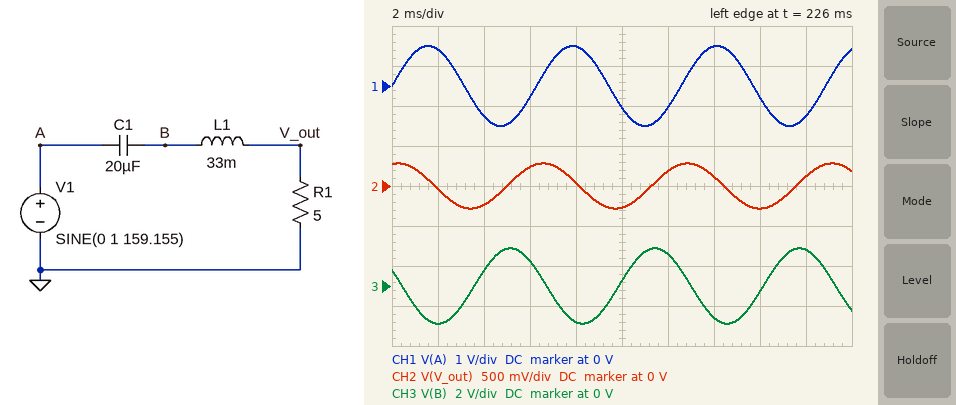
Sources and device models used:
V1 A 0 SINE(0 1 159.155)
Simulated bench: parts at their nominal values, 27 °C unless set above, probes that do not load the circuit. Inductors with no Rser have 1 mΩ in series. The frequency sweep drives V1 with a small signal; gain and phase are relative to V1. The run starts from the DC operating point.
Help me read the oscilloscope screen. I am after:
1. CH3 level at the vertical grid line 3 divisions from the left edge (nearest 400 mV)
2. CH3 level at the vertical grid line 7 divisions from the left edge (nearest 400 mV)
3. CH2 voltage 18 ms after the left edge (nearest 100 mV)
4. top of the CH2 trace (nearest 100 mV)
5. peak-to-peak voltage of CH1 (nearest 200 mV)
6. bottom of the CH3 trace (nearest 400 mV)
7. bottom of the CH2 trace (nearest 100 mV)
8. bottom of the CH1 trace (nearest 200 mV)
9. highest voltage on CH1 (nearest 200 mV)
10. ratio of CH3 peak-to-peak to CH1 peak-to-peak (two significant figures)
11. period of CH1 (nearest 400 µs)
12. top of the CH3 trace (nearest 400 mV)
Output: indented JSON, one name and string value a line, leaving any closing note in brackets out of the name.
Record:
{
  "CH3 level at the vertical grid line 3 divisions from the left edge": "1.2 V",
  "CH3 level at the vertical grid line 7 divisions from the left edge": "-1.6 V",
  "CH2 voltage 18 ms after the left edge": "100 mV",
  "top of the CH2 trace": "300 mV",
  "peak-to-peak voltage of CH1": "2.0 V",
  "bottom of the CH3 trace": "-2.0 V",
  "bottom of the CH2 trace": "-300 mV",
  "bottom of the CH1 trace": "-1.0 V",
  "highest voltage on CH1": "1.0 V",
  "ratio of CH3 peak-to-peak to CH1 peak-to-peak": "1.9",
  "period of CH1": "6.4 ms",
  "top of the CH3 trace": "2.0 V"
}
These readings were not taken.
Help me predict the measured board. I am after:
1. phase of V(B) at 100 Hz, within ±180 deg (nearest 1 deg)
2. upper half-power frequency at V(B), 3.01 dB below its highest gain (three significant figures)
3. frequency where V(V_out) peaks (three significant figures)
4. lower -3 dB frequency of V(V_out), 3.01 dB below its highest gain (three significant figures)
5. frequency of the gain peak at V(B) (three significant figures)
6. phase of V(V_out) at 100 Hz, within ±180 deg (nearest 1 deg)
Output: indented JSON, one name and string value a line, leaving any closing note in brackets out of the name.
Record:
{
  "phase of V(B) at 100 Hz, within ±180 deg": "162 deg",
  "upper half-power frequency at V(B), 3.01 dB below its highest gain": "210 Hz",
  "frequency where V(V_out) peaks": "196 Hz",
  "lower -3 dB frequency of V(V_out), 3.01 dB below its highest gain": "184 Hz",
  "frequency of the gain peak at V(B)": "197 Hz",
  "phase of V(V_out) at 100 Hz, within ±180 deg": "85 deg"
}
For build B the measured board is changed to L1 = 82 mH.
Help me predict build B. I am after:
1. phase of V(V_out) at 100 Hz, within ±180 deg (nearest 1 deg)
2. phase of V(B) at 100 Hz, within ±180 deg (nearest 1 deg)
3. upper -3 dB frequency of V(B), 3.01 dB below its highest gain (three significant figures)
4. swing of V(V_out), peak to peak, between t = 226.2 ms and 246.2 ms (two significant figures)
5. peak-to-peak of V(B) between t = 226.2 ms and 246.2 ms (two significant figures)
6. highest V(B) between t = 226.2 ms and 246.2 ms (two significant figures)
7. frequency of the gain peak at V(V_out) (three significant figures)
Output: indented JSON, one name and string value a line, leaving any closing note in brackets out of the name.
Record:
{
  "phase of V(V_out) at 100 Hz, within ±180 deg": "80 deg",
  "phase of V(B) at 100 Hz, within ±180 deg": "164 deg",
  "upper -3 dB frequency of V(B), 3.01 dB below its highest gain": "130 Hz",
  "swing of V(V_out), peak to peak, between t = 226.2 ms and 246.2 ms": "310 mV",
  "peak-to-peak of V(B) between t = 226.2 ms and 246.2 ms": "5.1 V",
  "highest V(B) between t = 226.2 ms and 246.2 ms": "2.5 V",
  "frequency of the gain peak at V(V_out)": "124 Hz"
}
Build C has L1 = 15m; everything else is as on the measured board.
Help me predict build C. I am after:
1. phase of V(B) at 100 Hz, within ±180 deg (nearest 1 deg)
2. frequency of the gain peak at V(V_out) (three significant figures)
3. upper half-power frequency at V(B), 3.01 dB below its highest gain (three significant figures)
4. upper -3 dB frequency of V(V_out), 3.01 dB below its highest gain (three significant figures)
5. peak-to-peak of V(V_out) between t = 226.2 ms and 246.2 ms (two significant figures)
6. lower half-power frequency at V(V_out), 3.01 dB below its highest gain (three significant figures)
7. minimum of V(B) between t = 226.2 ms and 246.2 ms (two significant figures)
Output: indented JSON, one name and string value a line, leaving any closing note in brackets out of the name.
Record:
{
  "phase of V(B) at 100 Hz, within ±180 deg": "148 deg",
  "frequency of the gain peak at V(V_out)": "291 Hz",
  "upper half-power frequency at V(B), 3.01 dB below its highest gain": "324 Hz",
  "upper -3 dB frequency of V(V_out), 3.01 dB below its highest gain": "318 Hz",
  "peak-to-peak of V(V_out) between t = 226.2 ms and 246.2 ms": "280 mV",
  "lower half-power frequency at V(V_out), 3.01 dB below its highest gain": "265 Hz",
  "minimum of V(B) between t = 226.2 ms and 246.2 ms": "-450 mV"
}
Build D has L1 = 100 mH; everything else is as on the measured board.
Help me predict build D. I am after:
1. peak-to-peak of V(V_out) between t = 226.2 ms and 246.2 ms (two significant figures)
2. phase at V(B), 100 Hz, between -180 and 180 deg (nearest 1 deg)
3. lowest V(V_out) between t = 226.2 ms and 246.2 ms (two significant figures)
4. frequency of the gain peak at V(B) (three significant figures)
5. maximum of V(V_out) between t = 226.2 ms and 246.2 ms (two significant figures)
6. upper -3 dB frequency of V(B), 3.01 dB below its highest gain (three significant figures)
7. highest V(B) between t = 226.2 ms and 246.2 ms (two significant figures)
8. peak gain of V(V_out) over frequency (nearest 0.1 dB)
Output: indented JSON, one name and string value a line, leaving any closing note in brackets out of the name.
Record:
{
  "peak-to-peak of V(V_out) between t = 226.2 ms and 246.2 ms": "200 mV",
  "phase at V(B), 100 Hz, between -180 and 180 deg": "159 deg",
  "lowest V(V_out) between t = 226.2 ms and 246.2 ms": "-100 mV",
  "frequency of the gain peak at V(B)": "113 Hz",
  "maximum of V(V_out) between t = 226.2 ms and 246.2 ms": "100 mV",
  "upper -3 dB frequency of V(B), 3.01 dB below its highest gain": "117 Hz",
  "highest V(B) between t = 226.2 ms and 246.2 ms": "2.0 V",
  "peak gain of V(V_out) over frequency": "0 dB"
}
